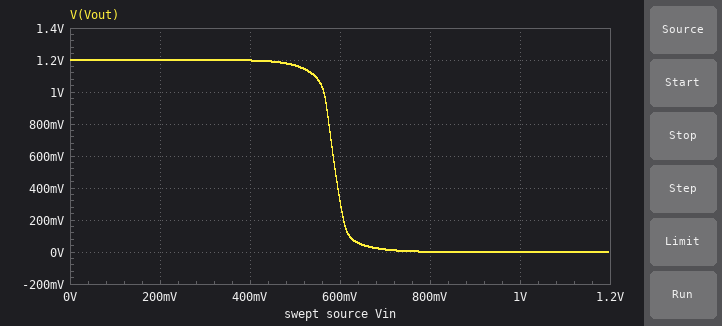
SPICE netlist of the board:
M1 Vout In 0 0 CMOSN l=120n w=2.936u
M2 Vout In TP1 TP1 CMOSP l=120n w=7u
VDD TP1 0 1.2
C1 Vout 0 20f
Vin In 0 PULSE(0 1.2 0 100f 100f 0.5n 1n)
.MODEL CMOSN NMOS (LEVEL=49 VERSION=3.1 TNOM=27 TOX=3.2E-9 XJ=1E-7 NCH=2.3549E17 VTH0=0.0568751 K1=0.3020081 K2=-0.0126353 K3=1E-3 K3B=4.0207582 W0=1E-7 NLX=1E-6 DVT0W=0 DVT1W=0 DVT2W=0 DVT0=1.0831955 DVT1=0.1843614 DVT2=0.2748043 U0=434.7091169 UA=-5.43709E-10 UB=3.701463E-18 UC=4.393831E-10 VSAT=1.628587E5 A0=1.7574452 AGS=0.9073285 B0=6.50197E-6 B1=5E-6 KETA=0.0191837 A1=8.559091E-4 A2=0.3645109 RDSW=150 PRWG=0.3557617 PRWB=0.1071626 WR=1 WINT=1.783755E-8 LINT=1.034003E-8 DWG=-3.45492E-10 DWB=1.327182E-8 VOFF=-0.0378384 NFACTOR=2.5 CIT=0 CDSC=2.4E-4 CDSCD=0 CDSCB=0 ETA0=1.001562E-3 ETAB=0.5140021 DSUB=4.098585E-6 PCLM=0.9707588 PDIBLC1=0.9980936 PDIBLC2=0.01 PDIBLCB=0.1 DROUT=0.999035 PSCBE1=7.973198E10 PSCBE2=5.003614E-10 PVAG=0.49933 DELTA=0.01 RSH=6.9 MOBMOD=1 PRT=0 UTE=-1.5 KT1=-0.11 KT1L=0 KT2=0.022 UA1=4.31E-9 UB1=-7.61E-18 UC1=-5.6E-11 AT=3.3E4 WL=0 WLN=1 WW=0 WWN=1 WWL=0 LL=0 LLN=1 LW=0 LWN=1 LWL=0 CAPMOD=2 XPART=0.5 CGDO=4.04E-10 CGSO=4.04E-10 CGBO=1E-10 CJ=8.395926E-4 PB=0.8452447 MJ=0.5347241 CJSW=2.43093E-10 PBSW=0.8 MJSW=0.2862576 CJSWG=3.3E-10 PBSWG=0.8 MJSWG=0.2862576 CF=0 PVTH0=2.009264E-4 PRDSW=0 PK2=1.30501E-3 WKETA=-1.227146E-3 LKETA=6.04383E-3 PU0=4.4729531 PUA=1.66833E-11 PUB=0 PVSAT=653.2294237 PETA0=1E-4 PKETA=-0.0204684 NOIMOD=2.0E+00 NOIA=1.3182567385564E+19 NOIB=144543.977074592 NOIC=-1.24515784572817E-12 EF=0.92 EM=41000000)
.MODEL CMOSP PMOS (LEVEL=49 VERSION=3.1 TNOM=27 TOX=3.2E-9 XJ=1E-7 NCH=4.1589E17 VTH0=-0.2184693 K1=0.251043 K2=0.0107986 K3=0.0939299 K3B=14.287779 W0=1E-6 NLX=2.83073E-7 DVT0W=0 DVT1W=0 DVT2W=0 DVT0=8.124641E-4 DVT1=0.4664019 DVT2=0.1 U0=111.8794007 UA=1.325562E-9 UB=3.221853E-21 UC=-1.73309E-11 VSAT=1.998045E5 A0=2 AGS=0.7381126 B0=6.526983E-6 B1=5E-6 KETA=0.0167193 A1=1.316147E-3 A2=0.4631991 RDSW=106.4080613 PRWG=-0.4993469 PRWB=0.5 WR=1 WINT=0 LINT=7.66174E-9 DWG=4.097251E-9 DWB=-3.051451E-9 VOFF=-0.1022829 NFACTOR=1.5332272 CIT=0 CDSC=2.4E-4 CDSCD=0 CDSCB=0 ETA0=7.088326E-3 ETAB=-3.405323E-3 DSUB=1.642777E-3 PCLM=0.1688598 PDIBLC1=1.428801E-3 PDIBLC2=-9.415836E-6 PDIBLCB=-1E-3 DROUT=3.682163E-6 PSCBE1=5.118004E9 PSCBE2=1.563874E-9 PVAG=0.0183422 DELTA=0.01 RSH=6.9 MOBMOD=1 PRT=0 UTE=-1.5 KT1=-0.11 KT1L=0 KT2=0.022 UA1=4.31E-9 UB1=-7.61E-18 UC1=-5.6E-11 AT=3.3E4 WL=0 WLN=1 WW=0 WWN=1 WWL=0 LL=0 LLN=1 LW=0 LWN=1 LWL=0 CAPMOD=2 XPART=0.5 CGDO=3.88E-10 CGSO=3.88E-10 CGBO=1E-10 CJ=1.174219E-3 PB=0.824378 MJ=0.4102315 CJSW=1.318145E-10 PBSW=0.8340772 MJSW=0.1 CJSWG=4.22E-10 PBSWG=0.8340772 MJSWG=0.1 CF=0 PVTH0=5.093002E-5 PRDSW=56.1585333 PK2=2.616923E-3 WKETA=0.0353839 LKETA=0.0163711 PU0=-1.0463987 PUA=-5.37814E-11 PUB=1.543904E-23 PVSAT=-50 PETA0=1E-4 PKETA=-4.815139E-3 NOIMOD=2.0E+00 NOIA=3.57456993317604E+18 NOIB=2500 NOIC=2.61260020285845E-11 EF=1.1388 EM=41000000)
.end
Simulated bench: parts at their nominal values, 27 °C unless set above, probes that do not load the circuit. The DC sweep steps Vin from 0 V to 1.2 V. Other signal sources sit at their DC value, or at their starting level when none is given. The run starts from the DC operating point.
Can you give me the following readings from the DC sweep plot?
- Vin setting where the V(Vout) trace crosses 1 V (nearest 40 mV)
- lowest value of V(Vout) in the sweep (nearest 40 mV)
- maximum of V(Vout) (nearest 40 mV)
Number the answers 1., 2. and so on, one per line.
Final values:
1. 560 mV
2. 0 V
3. 1.20 V
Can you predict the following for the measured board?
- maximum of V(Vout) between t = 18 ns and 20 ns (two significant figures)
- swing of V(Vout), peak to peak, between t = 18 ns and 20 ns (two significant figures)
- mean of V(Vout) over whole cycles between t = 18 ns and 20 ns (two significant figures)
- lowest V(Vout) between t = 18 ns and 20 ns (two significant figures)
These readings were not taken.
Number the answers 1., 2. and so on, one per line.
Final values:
1. 1.5 V
2. 1.8 V
3. 600 mV
4. -280 mV
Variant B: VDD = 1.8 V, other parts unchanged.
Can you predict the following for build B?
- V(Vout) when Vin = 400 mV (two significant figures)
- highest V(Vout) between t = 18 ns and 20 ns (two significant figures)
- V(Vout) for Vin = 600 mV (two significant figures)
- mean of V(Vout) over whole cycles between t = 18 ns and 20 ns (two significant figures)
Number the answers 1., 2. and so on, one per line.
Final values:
1. 1.8 V
2. 2.1 V
3. 1.7 V
4. 950 mV
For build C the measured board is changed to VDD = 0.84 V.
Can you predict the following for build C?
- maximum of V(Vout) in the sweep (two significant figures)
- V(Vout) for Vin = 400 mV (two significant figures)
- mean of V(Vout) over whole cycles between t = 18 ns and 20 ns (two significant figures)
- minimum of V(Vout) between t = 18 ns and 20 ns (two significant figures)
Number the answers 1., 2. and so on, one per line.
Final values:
1. 840 mV
2. 810 mV
3. 390 mV
4. -250 mV
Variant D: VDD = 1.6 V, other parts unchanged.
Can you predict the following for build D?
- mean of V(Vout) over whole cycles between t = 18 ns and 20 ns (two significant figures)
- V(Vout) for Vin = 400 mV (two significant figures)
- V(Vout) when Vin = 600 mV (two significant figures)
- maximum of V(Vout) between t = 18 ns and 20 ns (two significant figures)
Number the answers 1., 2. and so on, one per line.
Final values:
1. 820 mV
2. 1.6 V
3. 1.5 V
4. 1.9 V
